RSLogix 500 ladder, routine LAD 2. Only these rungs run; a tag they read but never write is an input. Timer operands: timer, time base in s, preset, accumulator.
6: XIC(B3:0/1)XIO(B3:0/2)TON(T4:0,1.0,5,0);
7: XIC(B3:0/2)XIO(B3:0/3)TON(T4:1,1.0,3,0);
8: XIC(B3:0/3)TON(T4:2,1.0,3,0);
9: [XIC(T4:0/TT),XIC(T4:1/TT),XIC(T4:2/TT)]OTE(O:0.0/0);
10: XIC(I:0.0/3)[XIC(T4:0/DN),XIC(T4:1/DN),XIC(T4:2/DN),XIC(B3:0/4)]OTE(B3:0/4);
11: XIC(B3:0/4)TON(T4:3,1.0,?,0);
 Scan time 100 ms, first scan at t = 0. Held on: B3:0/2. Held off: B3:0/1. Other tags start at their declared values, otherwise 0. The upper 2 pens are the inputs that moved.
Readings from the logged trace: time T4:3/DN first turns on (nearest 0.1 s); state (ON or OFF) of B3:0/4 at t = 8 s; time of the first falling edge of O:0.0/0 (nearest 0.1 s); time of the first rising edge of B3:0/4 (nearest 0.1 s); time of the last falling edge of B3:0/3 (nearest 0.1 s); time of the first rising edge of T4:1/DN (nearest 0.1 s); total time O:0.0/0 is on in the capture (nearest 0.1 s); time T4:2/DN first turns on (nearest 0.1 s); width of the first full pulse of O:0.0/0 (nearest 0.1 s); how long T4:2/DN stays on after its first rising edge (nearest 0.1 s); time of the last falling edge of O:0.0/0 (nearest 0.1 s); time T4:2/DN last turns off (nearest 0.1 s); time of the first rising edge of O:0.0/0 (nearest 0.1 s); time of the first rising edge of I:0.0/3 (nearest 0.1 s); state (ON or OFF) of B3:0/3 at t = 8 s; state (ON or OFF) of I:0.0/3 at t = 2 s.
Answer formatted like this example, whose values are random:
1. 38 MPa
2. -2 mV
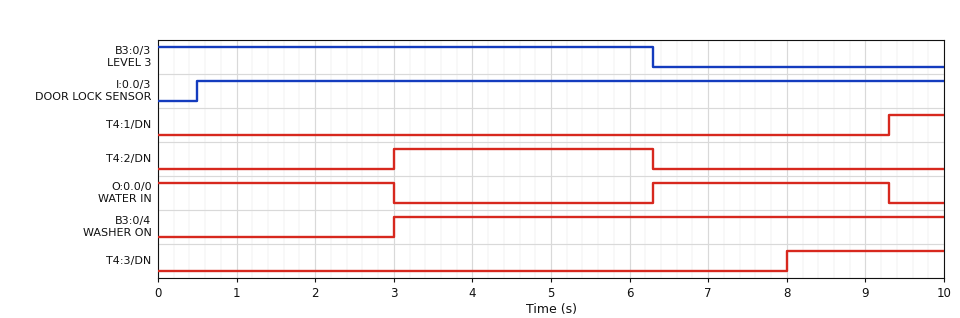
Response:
1. 8.0 s
2. ON
3. 3.0 s
4. 3.0 s
5. 6.3 s
6. 9.3 s
7. 6.0 s
8. 3.0 s
9. 3.0 s
10. 3.3 s
11. 9.3 s
12. 6.3 s
13. 6.3 s
14. 0.5 s
15. OFF
16. ON
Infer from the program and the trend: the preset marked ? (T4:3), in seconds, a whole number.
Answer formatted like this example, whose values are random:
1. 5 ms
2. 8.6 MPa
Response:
1. 5 s
